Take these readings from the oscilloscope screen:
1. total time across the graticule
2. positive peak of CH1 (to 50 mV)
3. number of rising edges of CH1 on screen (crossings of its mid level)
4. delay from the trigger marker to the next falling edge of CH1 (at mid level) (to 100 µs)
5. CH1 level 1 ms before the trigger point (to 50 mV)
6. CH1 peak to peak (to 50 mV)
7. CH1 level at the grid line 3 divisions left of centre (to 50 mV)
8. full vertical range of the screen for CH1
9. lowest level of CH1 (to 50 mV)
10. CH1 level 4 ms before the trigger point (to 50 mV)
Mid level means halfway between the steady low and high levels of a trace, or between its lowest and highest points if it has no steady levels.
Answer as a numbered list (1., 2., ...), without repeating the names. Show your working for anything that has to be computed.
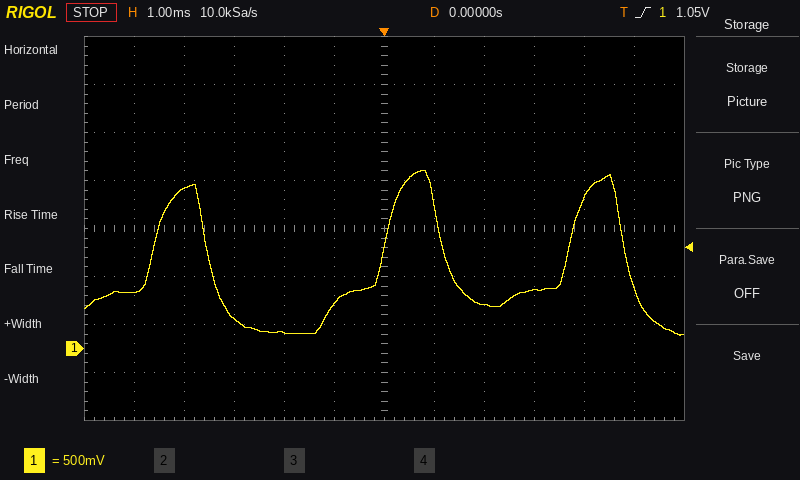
1. 12 ms
2. 1.85 V
3. 3
4. 1.2 ms
5. 450 mV
6. 1.85 V − (150 mV) = 1.70 V
7. 300 mV
8. 4 V
9. 150 mV
10. 1.65 V
